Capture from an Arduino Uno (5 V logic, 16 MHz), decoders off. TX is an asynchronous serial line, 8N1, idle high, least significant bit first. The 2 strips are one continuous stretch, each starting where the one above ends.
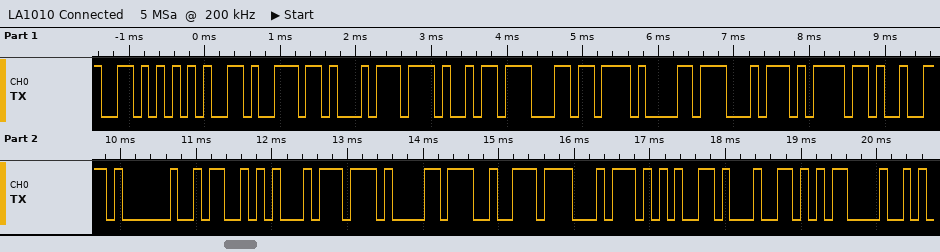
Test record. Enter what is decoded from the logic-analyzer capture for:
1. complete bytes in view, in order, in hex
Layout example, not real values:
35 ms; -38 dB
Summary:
0x56 0x65 0x6E 0x74 0x69 0x6C 0x61 0x74 0x6F 0x72 0x20 0x53 0x74 0x61 0x72 0x74 0x65 0x64 0x0D
